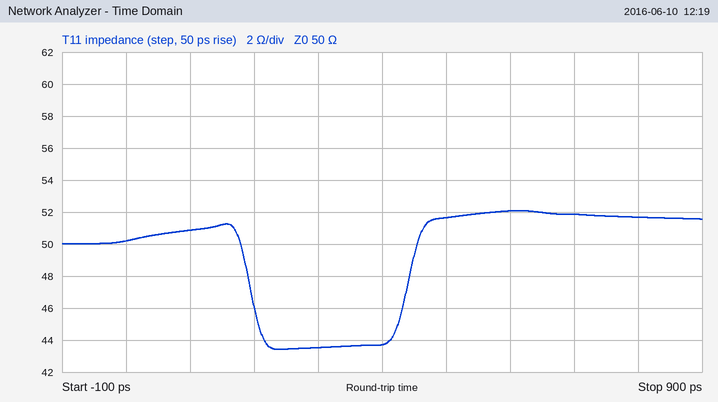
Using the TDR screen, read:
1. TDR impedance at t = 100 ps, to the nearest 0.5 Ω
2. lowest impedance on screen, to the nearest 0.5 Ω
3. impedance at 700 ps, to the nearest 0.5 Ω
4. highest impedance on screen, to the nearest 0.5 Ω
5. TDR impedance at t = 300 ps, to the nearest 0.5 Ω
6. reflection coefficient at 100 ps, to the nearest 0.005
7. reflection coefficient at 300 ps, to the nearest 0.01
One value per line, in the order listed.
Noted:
51.0 Ω
43.5 Ω
52.0 Ω
52.0 Ω
43.5 Ω
+0.010
-0.07
